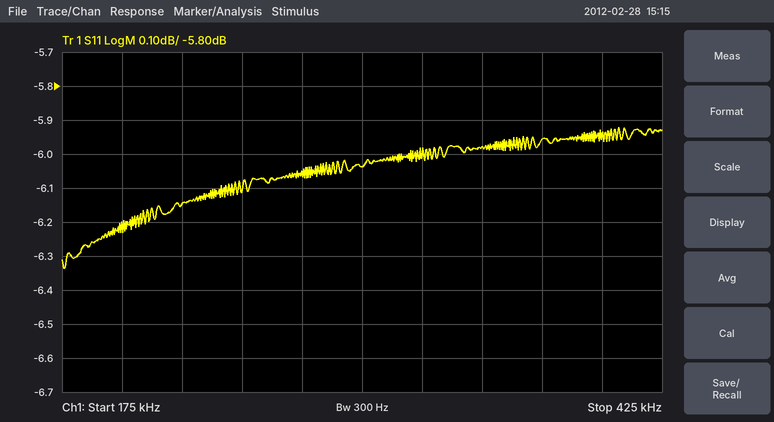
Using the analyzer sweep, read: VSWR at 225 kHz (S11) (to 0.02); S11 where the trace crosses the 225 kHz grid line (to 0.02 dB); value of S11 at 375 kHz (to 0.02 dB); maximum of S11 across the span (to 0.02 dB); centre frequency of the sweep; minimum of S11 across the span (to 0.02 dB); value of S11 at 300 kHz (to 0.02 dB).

2.94
-6.14 dB
-5.96 dB
-5.92 dB
300 kHz
-6.34 dB
-6.04 dB
